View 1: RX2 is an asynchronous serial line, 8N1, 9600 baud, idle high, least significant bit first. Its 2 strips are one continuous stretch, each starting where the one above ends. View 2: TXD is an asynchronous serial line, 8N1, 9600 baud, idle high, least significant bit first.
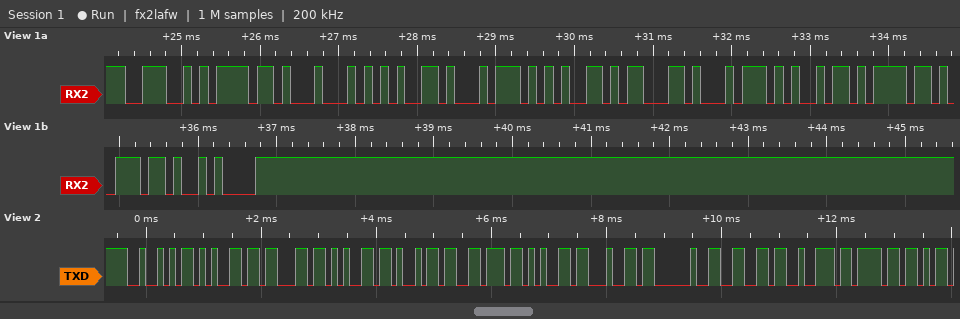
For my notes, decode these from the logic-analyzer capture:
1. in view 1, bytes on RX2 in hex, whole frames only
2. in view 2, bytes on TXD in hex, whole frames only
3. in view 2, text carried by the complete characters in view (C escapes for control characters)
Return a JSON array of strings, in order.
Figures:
["4E 6F 44 65 74 65 63 74 69 6F 6E 0A", "52 65 63 65 69 76 65 64 20 66 72 6F", "\"Received fro\""]
